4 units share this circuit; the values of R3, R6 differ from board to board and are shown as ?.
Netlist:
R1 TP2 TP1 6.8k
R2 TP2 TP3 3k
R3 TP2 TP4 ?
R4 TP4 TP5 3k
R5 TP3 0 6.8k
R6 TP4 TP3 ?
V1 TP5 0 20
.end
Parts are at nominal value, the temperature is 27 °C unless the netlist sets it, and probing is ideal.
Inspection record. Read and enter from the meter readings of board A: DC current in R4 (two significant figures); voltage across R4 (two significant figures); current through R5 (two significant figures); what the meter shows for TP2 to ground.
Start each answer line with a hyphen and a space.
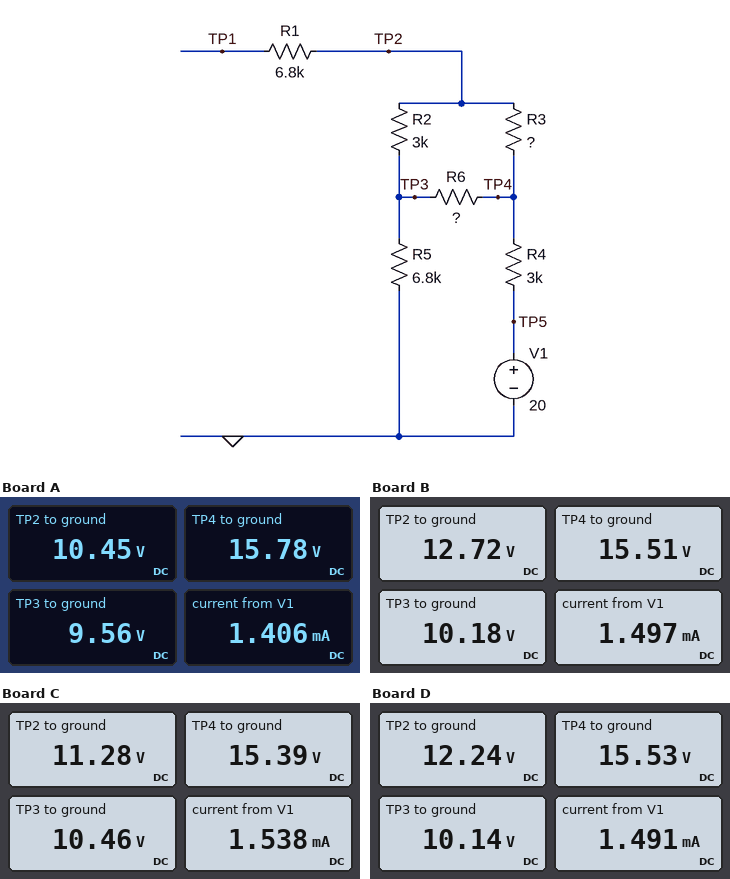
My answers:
- 1.4 mA
- 4.2 V
- 1.4 mA
- 10.45 V
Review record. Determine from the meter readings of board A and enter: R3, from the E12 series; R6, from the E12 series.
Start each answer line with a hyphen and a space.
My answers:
- 18 kΩ
- 5.6 kΩ
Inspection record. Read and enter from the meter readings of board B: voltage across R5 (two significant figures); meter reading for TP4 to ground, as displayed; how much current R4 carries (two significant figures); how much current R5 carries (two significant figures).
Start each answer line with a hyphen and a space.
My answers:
- 10 V
- 15.51 V
- 1.5 mA
- 1.5 mA
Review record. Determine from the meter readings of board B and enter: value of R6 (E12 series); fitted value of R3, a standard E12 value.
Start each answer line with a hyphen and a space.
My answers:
- 8.2 kΩ
- 3.3 kΩ
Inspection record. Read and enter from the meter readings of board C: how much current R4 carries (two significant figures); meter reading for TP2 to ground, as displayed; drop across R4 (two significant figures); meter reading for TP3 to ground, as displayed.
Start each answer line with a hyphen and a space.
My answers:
- 1.5 mA
- 11.28 V
- 4.6 V
- 10.46 V
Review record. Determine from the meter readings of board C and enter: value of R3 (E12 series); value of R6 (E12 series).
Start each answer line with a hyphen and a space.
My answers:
- 15 kΩ
- 3.9 kΩ
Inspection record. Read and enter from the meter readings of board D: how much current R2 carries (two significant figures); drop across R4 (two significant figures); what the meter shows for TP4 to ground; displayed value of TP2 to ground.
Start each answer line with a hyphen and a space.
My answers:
- 700 µA
- 4.5 V
- 15.53 V
- 12.24 V
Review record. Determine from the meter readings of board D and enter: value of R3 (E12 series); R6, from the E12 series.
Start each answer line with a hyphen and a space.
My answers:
- 4.7 kΩ
- 6.8 kΩ
